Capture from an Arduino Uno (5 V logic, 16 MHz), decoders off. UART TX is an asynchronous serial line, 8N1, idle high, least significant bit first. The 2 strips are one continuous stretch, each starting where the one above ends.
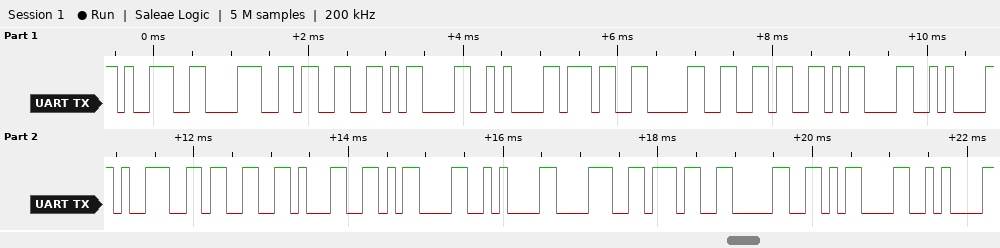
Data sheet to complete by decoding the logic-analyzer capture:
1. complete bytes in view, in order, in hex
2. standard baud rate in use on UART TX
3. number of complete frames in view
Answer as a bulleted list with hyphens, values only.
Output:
- 0x39 0x38 0x33 0x0D 0x0A 0x37 0x30 0x36 0x0D 0x0A 0x39 0x33 0x31 0x0D 0x0A 0x38 0x37 0x30 0x0D 0x0A
- 9600 baud
- 20
